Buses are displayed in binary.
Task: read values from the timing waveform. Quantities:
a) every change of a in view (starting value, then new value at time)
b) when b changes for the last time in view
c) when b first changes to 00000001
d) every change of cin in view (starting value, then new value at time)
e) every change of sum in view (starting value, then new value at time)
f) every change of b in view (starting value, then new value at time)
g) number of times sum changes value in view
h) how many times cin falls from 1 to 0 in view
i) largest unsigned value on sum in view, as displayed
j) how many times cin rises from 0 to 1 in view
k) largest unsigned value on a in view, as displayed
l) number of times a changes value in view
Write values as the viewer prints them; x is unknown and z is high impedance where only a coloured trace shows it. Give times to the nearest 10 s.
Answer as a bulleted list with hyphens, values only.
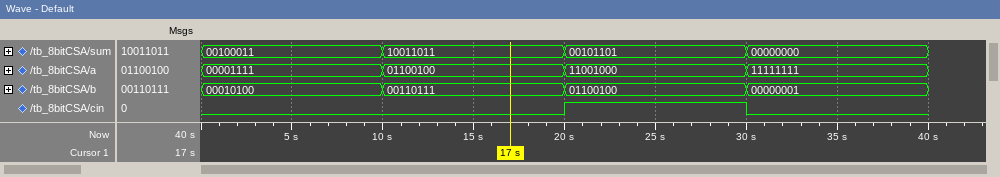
- 00001111, 01100100 at 10 s, 11001000 at 20 s, 11111111 at 30 s
- 30 s
- 30 s
- 0, 1 at 20 s, 0 at 30 s
- 00100011, 10011011 at 10 s, 00101101 at 20 s, 00000000 at 30 s
- 00010100, 00110111 at 10 s, 01100100 at 20 s, 00000001 at 30 s
- 3
- 1
- 10011011
- 1
- 11111111
- 3
